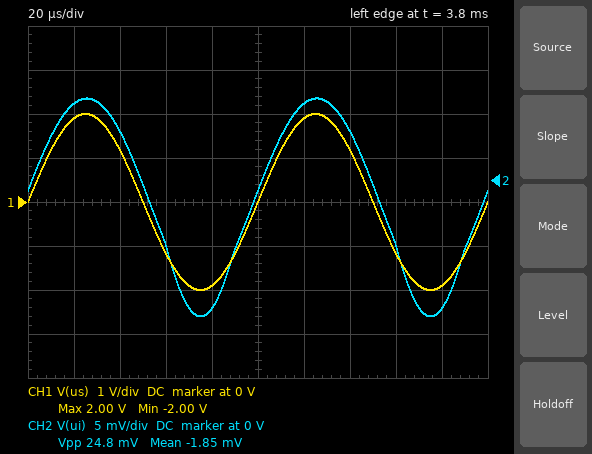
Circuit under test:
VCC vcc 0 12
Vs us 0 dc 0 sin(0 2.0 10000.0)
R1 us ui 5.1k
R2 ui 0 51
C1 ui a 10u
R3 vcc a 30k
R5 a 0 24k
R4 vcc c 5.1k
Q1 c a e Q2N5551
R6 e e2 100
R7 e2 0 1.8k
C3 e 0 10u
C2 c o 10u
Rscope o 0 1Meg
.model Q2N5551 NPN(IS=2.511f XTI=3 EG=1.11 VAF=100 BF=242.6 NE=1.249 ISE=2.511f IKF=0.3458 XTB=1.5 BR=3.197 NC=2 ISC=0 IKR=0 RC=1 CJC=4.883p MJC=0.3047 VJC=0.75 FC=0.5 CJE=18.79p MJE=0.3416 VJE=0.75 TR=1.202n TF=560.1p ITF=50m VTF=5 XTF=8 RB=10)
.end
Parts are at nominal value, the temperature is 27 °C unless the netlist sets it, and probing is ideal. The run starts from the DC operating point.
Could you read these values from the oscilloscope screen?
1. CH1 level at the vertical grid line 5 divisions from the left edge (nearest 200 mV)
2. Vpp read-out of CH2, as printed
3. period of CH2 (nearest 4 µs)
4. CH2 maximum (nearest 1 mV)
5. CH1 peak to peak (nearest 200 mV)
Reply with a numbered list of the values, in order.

1. 0 V
2. 24.8 mV
3. 100 µs
4. 9 mV
5. 4.0 V
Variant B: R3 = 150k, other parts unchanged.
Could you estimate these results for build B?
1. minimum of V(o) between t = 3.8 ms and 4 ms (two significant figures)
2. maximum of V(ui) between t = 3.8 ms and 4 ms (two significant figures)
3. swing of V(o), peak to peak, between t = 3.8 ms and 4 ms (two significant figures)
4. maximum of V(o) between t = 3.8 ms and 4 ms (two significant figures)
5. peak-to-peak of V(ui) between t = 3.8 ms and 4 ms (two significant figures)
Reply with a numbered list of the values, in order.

1. -2.0 V
2. 20 mV
3. 3.4 V
4. 1.4 V
5. 39 mV
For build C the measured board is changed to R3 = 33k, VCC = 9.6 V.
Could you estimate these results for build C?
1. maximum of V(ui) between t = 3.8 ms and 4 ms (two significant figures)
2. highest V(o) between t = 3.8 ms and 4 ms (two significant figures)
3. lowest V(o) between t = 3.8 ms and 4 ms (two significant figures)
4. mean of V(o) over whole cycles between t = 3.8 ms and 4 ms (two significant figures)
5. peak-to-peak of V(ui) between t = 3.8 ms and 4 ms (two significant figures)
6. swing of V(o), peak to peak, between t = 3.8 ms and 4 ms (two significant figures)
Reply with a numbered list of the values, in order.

1. 10 mV
2. 2.3 V
3. -58 mV
4. 550 mV
5. 28 mV
6. 2.4 V
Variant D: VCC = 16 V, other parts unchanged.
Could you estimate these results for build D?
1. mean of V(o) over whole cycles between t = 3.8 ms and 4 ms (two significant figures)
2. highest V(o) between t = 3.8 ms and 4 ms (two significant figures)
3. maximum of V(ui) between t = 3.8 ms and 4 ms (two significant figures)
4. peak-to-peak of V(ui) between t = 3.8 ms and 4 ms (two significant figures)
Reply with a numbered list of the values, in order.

1. 320 mV
2. 2.0 V
3. 8.4 mV
4. 22 mV
